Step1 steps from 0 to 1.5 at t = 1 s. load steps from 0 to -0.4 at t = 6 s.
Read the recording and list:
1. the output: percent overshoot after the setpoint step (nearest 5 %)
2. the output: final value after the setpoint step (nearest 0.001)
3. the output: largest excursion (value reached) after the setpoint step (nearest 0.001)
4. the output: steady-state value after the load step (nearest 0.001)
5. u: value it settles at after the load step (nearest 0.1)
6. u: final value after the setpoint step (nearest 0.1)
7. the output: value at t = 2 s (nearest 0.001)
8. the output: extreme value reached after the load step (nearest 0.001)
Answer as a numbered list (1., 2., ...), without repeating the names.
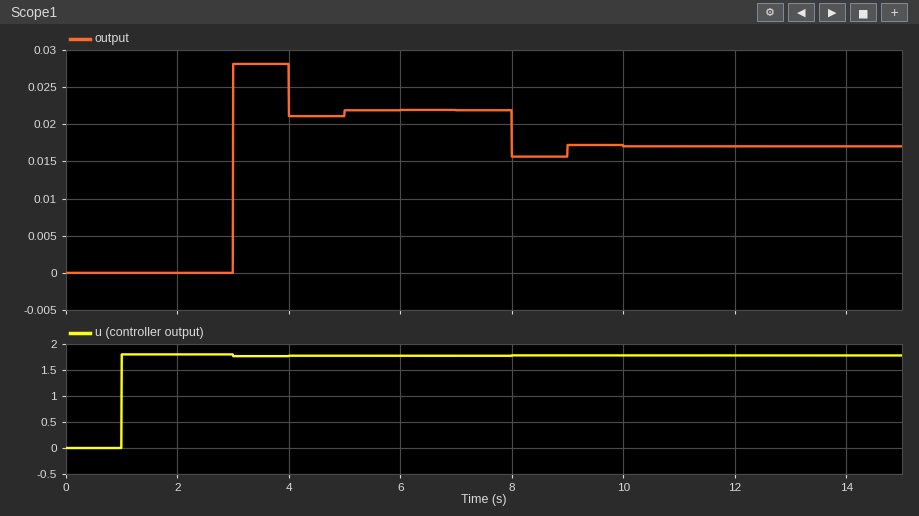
1. 30 %
2. 0.022
3. 0.028
4. 0.017
5. 1.8
6. 1.8
7. 0.000
8. 0.016
